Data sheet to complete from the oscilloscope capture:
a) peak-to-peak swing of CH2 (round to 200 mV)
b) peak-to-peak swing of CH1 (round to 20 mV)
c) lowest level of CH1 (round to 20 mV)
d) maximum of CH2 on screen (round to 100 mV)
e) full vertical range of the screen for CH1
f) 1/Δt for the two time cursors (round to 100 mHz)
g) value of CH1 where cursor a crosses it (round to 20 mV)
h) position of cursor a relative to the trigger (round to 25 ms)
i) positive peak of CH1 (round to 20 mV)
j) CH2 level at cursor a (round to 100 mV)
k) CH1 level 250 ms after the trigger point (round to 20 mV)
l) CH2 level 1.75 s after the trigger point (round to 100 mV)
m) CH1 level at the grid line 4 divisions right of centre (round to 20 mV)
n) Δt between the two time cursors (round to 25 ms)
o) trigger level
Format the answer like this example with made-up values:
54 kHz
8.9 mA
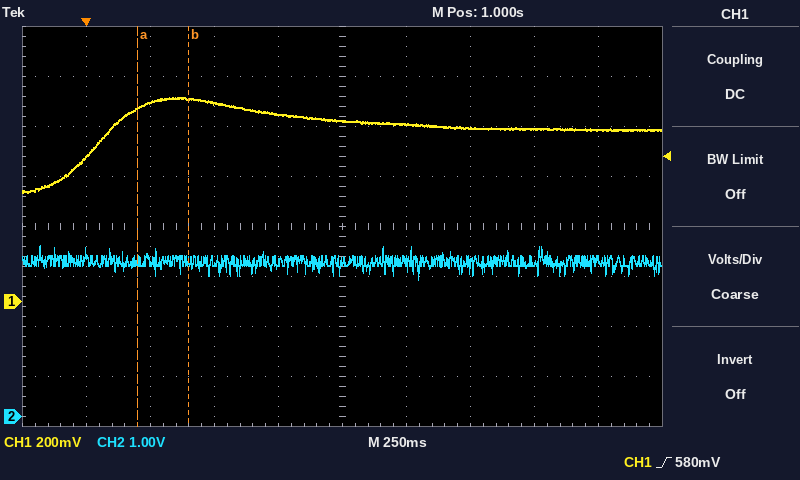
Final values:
600 mV
380 mV
440 mV
3.4 V
1.6 V
5.0 Hz
780 mV
+200 ms
820 mV
3.1 V
800 mV
3.1 V
680 mV
200 ms
580 mV
